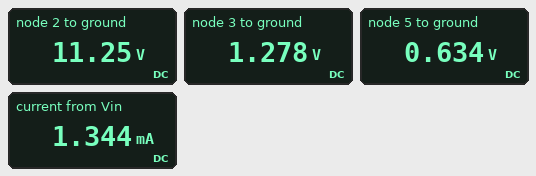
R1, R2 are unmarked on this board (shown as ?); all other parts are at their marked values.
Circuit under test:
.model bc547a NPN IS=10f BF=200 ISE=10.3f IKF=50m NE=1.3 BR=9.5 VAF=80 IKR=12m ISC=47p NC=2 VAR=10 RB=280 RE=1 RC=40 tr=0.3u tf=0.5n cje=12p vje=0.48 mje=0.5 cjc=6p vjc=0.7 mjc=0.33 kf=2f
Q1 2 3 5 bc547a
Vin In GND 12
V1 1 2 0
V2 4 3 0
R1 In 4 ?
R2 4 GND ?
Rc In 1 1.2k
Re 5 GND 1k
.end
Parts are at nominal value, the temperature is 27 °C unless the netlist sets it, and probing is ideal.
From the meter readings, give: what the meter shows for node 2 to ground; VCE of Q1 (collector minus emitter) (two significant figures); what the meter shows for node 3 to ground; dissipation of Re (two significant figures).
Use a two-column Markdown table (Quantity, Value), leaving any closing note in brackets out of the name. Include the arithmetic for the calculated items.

| Quantity | Value |
|---|---|
| what the meter shows for node 2 to ground | 11.25 V |
| VCE of Q1 (collector minus emitter) | 11.25 V - 634 mV = 11 V |
| what the meter shows for node 3 to ground | 1.278 V |
| dissipation of Re | (634 mV)^2 / 1 kΩ = 400 µW |
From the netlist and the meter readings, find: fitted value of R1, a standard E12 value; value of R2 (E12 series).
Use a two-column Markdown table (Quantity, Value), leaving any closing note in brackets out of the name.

| Quantity | Value |
|---|---|
| fitted value of R1, a standard E12 value | 15 kΩ |
| value of R2 | 1.8 kΩ |
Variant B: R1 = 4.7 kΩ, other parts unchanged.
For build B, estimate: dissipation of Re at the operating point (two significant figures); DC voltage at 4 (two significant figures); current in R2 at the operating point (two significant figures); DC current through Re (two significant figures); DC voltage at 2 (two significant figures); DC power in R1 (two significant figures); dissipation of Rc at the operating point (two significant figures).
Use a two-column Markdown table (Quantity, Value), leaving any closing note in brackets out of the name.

| Quantity | Value |
|---|---|
| dissipation of Re at the operating point | 6.8 mW |
| DC voltage at 4 | 3.3 V |
| current in R2 at the operating point | 1.8 mA |
| DC current through Re | 2.6 mA |
| DC voltage at 2 | 8.9 V |
| DC power in R1 | 16 mW |
| dissipation of Rc at the operating point | 8.0 mW |
